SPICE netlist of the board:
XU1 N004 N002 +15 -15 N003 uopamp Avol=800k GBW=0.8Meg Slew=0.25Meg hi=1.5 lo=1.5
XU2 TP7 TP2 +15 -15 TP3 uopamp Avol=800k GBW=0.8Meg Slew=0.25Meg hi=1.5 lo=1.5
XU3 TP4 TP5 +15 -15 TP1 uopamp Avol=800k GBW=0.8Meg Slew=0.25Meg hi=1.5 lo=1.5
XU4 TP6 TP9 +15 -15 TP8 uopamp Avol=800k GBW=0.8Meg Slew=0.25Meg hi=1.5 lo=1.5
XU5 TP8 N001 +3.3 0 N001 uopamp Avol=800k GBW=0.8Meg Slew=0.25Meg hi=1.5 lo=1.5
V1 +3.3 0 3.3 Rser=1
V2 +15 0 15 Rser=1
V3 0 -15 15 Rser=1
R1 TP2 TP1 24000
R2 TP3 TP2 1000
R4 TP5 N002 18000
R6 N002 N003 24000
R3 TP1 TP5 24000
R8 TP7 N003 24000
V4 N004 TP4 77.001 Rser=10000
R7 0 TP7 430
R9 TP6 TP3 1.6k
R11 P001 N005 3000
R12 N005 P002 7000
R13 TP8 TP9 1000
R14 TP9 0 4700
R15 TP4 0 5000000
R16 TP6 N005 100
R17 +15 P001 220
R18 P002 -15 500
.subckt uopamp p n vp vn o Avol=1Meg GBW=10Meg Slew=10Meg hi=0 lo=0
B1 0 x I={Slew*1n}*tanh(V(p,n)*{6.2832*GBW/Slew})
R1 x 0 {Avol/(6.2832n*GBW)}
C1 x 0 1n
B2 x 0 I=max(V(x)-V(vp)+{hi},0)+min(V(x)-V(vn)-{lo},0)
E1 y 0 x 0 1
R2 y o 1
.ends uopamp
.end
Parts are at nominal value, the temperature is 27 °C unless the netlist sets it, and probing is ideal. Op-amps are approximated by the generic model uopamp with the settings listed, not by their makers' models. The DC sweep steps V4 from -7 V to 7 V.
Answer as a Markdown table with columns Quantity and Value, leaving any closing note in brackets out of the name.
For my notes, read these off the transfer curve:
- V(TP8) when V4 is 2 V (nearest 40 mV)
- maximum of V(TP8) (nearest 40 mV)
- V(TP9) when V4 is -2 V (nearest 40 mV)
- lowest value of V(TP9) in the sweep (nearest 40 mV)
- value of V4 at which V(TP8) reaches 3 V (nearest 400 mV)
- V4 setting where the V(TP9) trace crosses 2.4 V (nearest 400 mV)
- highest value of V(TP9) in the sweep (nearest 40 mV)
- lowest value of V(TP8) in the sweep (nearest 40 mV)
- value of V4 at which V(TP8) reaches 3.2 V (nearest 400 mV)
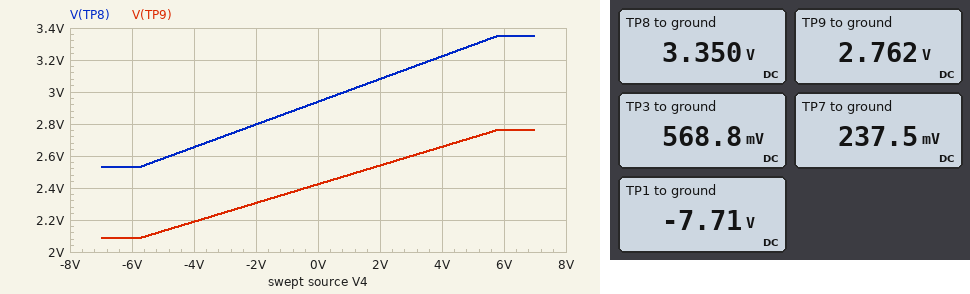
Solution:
| Quantity | Value |
|---|---|
| V(TP8) when V4 is 2 V | 3.08 V |
| maximum of V(TP8) | 3.36 V |
| V(TP9) when V4 is -2 V | 2.32 V |
| lowest value of V(TP9) in the sweep | 2.08 V |
| value of V4 at which V(TP8) reaches 3 V | 800 mV |
| V4 setting where the V(TP9) trace crosses 2.4 V | -400 mV |
| highest value of V(TP9) in the sweep | 2.76 V |
| lowest value of V(TP8) in the sweep | 2.52 V |
| value of V4 at which V(TP8) reaches 3.2 V | 3.6 V |
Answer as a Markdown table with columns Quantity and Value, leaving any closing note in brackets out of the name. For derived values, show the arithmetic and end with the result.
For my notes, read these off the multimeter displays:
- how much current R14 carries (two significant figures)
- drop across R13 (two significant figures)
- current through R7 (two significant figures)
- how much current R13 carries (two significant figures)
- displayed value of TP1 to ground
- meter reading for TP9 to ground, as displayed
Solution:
| Quantity | Value |
|---|---|
| how much current R14 carries | (2.762 V) / 4.7 kΩ = 590 µA |
| drop across R13 | 3.35 V - 2.762 V = 590 mV |
| current through R7 | (237.5 mV) / 430 Ω = 550 µA |
| how much current R13 carries | (3.35 V - 2.762 V) / 1 kΩ = 590 µA |
| displayed value of TP1 to ground | -7.71 V |
| meter reading for TP9 to ground, as displayed | 2.762 V |
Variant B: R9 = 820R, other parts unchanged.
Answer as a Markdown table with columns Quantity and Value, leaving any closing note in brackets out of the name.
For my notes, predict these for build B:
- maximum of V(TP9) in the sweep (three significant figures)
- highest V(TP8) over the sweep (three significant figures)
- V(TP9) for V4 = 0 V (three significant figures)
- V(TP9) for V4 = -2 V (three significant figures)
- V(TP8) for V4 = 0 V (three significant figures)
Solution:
| Quantity | Value |
|---|---|
| maximum of V(TP9) in the sweep | 1.97 V |
| highest V(TP8) over the sweep | 2.39 V |
| V(TP9) for V4 = 0 V | 1.55 V |
| V(TP9) for V4 = -2 V | 1.40 V |
| V(TP8) for V4 = 0 V | 1.88 V |
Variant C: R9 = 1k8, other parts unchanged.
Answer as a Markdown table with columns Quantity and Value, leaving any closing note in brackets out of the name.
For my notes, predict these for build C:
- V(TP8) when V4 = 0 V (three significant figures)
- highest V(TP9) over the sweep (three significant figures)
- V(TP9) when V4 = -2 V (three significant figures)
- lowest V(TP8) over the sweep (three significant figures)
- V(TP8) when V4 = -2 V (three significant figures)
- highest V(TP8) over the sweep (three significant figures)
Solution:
| Quantity | Value |
|---|---|
| V(TP8) when V4 = 0 V | 3.15 V |
| highest V(TP9) over the sweep | 2.92 V |
| V(TP9) when V4 = -2 V | 2.48 V |
| lowest V(TP8) over the sweep | 2.76 V |
| V(TP8) when V4 = -2 V | 3.01 V |
| highest V(TP8) over the sweep | 3.54 V |
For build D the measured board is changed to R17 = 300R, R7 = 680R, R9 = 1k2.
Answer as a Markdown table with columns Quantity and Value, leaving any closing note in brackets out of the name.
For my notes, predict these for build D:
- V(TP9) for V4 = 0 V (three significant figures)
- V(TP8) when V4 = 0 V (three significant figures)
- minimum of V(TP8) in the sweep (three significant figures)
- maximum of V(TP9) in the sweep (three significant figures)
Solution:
| Quantity | Value |
|---|---|
| V(TP9) for V4 = 0 V | 1.95 V |
| V(TP8) when V4 = 0 V | 2.36 V |
| minimum of V(TP8) in the sweep | 1.79 V |
| maximum of V(TP9) in the sweep | 2.42 V |
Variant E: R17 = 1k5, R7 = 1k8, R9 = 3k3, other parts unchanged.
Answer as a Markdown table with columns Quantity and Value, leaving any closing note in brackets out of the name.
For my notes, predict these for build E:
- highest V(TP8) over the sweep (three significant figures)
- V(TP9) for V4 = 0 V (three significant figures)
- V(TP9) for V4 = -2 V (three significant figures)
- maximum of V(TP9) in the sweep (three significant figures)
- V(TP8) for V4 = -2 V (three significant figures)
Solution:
| Quantity | Value |
|---|---|
| highest V(TP8) over the sweep | 3.16 V |
| V(TP9) for V4 = 0 V | 1.99 V |
| V(TP9) for V4 = -2 V | 1.78 V |
| maximum of V(TP9) in the sweep | 2.60 V |
| V(TP8) for V4 = -2 V | 2.16 V |
